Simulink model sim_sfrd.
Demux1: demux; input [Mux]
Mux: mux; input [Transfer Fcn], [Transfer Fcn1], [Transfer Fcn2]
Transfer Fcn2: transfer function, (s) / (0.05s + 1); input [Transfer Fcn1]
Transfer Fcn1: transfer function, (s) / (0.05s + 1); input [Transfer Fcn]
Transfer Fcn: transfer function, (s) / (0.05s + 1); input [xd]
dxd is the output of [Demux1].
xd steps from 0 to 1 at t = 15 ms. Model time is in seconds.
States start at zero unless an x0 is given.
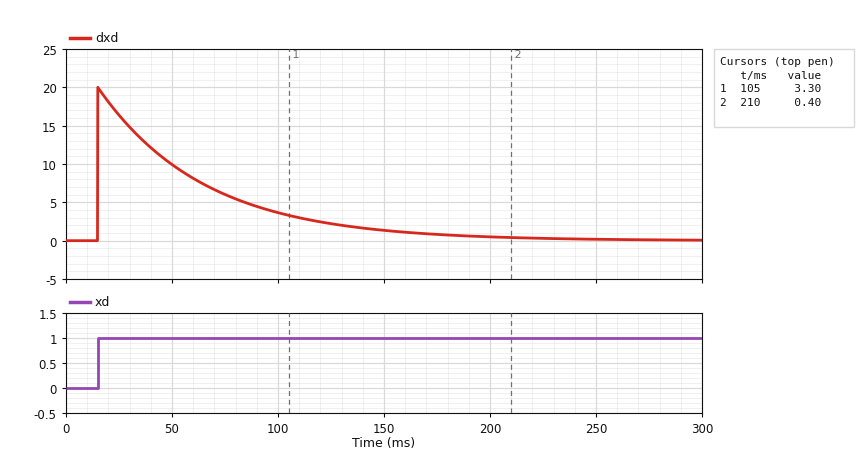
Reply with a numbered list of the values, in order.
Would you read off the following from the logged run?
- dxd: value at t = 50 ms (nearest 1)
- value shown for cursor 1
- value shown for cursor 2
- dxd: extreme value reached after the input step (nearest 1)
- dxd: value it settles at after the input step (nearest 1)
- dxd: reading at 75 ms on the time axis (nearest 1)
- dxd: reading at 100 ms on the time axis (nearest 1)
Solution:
1. 10
2. 3.30
3. 0.40
4. 20
5. 0
6. 6
7. 4
